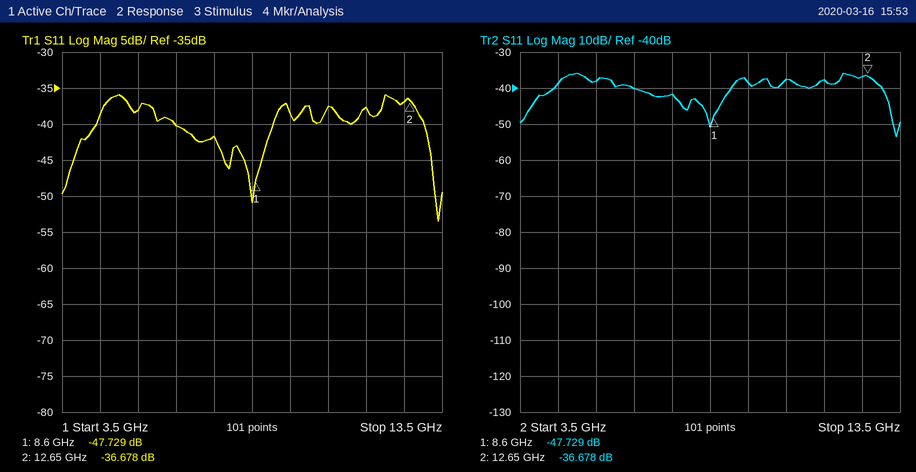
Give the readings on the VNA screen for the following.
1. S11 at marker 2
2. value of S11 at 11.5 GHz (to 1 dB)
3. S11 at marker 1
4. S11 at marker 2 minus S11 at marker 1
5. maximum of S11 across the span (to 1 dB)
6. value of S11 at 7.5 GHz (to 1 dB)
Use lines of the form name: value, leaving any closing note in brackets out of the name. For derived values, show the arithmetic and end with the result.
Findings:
S11 at marker 2: -36.678 dB
value of S11 at 11.5 GHz: -38 dB
S11 at marker 1: -47.729 dB
S11 at marker 2 minus S11 at marker 1: -36.678 − (-47.729) = 11.051 dB
maximum of S11 across the span: -36 dB
value of S11 at 7.5 GHz: -42 dB
